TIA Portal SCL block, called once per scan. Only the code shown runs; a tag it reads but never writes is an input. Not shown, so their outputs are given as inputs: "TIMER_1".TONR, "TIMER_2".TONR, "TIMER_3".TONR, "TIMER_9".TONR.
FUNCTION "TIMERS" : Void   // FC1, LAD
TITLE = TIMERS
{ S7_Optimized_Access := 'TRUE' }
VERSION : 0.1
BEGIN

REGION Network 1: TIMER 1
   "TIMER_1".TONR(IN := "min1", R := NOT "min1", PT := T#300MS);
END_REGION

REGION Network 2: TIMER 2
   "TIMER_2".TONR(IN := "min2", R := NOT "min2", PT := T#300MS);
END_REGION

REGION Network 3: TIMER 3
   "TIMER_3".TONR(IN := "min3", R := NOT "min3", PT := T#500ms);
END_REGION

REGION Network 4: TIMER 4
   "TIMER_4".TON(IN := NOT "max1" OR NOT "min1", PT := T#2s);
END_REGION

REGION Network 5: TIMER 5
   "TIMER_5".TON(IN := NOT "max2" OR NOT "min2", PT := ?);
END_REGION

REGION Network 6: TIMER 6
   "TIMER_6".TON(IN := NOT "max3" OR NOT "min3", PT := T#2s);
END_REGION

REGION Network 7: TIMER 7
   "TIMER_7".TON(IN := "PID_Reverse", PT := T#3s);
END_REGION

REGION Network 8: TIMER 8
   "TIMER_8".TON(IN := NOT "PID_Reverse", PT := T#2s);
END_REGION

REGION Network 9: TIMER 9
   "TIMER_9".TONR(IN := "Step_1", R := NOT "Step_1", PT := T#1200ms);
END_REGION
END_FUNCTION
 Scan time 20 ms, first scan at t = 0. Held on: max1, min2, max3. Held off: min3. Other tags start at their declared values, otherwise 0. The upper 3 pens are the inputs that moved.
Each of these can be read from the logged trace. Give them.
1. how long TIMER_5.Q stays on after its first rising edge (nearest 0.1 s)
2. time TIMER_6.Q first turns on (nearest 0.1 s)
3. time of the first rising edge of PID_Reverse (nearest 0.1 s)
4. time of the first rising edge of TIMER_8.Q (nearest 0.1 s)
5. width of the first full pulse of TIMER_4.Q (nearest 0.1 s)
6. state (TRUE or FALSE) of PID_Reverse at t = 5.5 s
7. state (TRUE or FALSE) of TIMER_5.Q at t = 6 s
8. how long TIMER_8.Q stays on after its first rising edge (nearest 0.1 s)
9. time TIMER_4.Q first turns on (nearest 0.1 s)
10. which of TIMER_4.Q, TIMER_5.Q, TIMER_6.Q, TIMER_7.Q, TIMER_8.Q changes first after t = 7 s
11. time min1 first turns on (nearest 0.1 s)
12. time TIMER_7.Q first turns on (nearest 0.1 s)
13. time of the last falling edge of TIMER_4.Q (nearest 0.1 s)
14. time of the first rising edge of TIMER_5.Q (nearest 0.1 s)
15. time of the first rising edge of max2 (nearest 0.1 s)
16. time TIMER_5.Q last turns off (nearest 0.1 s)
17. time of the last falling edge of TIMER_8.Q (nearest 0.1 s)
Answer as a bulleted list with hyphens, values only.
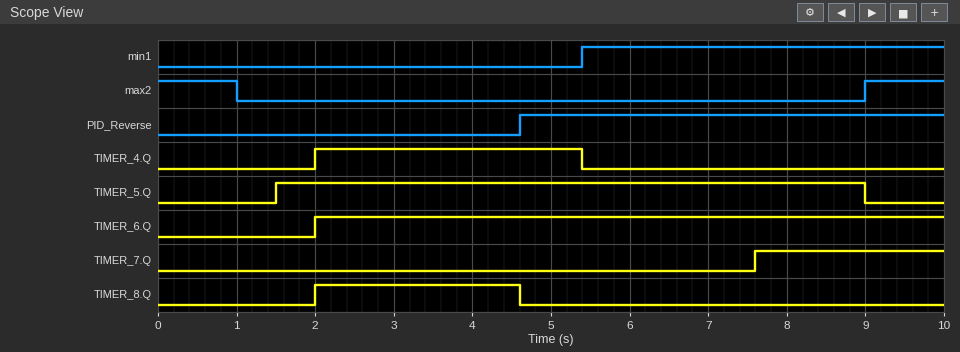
- 7.5 s
- 2.0 s
- 4.6 s
- 2.0 s
- 3.4 s
- TRUE
- TRUE
- 2.6 s
- 2.0 s
- TIMER_7.Q
- 5.4 s
- 7.6 s
- 5.4 s
- 1.5 s
- 9.0 s
- 9.0 s
- 4.6 s
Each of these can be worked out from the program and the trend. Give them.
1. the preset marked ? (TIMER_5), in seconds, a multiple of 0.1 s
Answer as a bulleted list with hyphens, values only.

- 0.5 s
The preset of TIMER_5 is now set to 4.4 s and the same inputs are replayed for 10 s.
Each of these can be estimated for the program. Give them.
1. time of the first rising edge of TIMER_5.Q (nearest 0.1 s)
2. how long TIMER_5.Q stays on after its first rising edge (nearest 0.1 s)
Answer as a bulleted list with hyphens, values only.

- 5.4 s
- 3.6 s
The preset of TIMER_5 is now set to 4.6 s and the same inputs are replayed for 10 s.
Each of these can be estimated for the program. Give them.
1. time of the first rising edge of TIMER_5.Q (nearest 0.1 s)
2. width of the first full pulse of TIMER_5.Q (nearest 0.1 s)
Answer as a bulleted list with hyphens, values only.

- 5.6 s
- 3.4 s
